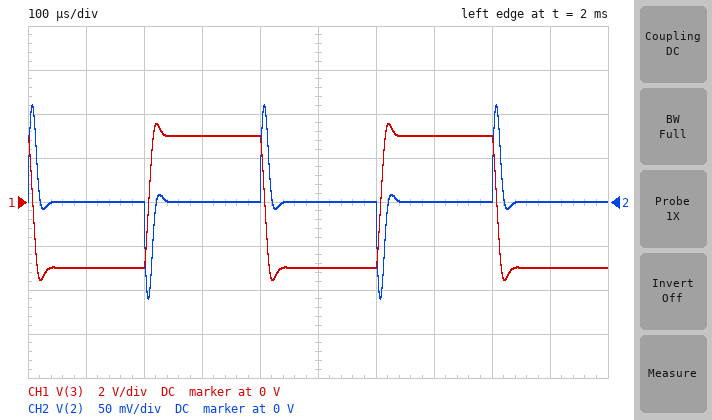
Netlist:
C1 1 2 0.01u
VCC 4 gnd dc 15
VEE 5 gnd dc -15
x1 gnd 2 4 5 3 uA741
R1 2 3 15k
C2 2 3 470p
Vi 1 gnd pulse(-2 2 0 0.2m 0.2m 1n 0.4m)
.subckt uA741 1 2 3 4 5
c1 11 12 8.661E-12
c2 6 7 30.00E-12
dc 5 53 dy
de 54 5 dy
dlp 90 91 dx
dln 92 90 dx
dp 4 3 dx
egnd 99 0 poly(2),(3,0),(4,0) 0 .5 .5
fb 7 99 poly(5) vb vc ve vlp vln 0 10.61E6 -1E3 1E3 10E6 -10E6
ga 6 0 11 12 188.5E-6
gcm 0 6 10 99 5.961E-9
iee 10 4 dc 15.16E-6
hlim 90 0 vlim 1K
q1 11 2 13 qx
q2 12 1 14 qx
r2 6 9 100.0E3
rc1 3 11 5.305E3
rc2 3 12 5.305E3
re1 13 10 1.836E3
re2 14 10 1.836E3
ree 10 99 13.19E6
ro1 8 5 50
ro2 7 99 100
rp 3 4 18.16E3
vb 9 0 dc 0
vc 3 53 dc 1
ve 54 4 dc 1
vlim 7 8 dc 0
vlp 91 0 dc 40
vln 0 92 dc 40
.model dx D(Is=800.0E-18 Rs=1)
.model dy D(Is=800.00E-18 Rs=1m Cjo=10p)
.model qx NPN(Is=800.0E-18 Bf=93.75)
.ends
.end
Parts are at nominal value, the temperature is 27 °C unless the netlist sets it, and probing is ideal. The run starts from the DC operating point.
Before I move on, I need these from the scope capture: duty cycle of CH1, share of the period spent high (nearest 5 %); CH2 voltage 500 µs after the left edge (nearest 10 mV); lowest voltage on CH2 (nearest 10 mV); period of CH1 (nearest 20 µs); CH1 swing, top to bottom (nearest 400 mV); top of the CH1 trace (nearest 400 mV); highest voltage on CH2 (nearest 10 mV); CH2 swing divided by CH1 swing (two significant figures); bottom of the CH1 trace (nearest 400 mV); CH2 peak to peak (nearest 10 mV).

50 %
0 V
-110 mV
400 µs
7.2 V
3.6 V
110 mV
0.031
-3.6 V
220 mV
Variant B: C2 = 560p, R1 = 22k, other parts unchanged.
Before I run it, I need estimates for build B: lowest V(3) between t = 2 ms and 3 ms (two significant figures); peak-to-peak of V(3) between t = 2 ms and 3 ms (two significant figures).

-4.4 V
8.8 V
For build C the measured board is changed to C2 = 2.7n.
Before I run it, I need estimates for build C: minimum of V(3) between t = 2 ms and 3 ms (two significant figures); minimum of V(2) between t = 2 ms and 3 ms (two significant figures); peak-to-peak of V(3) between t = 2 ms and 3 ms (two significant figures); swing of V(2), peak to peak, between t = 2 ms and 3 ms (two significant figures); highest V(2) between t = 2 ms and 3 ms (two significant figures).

-3.0 V
-23 mV
5.9 V
46 mV
23 mV
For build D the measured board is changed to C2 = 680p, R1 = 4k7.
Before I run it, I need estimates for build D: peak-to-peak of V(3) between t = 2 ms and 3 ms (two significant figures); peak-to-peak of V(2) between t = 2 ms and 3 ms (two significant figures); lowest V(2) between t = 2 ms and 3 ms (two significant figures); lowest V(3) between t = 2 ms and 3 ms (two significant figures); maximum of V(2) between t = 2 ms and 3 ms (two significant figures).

2.4 V
120 mV
-59 mV
-1.2 V
59 mV
